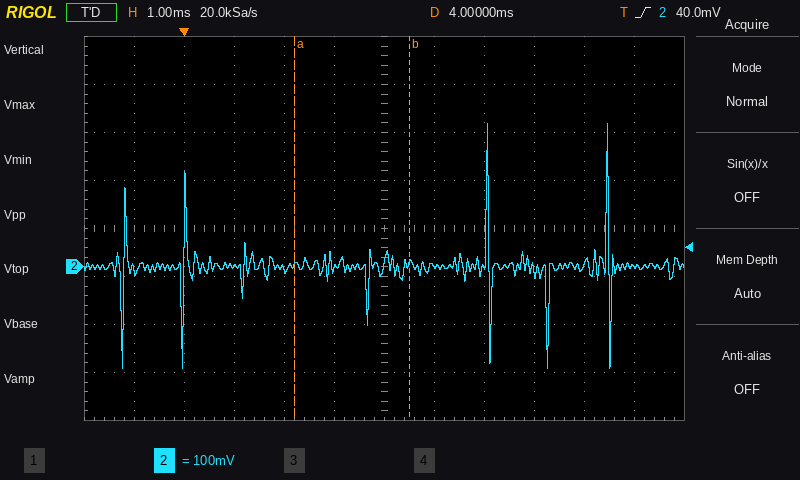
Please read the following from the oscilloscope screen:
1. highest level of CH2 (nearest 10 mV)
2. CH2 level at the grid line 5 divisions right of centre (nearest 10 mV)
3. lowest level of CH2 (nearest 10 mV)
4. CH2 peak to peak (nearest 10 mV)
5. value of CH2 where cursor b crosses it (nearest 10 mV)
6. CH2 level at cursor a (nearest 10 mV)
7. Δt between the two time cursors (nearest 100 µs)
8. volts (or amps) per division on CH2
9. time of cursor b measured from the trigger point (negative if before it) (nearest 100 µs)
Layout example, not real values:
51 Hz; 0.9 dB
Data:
300 mV; 0 mV; -210 mV; 510 mV; 10 mV; 0 mV; 2.3 ms; 100 mV; +4.5 ms
